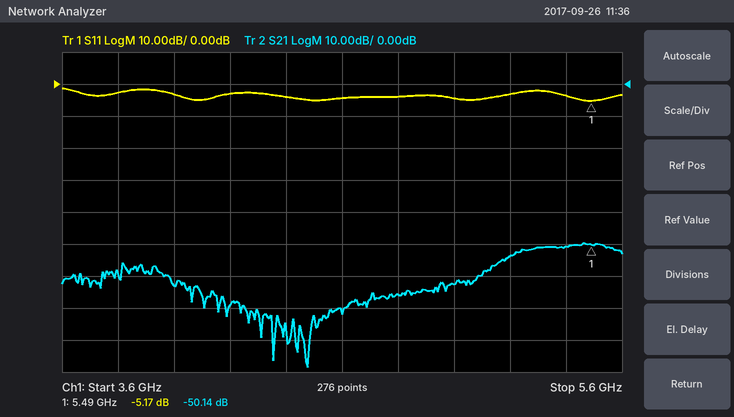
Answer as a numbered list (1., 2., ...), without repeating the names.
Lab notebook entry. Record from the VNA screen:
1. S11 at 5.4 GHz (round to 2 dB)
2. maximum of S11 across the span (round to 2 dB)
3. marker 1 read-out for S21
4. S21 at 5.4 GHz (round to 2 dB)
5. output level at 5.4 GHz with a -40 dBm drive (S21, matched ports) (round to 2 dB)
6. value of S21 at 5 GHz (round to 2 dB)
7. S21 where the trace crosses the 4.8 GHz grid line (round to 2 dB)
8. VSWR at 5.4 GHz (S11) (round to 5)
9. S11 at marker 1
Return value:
1. -4 dB
2. -2 dB
3. -50.14 dB
4. -50 dB
5. -90 dBm
6. -62 dB
7. -66 dB
8. 5
9. -5.17 dB
